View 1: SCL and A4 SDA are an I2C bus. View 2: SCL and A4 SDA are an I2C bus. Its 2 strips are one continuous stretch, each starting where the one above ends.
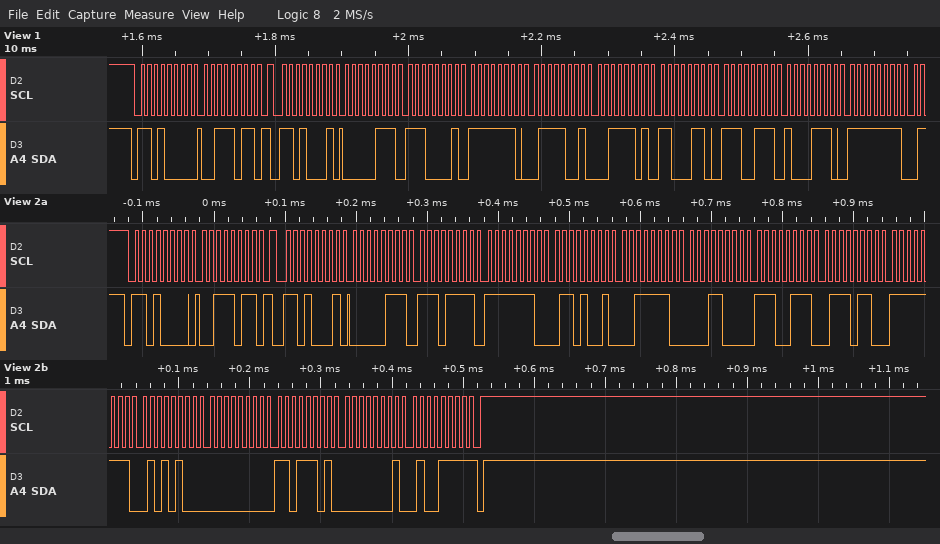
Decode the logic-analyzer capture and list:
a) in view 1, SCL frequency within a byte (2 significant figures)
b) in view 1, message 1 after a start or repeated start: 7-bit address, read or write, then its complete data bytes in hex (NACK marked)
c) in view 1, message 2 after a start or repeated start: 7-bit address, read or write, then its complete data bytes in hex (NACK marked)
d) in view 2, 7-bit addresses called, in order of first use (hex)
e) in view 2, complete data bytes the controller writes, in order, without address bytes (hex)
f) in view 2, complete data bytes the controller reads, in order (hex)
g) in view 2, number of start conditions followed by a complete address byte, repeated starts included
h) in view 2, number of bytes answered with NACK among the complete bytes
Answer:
100 kHz
0x68 write: 3B
0x68 read: 07 E1 FE 79 3D C6 E7 8E FF
0x68
3B
07 EF FE 69 3E 18 E7 76 FF 54 00 DD 01 4F
2
1
